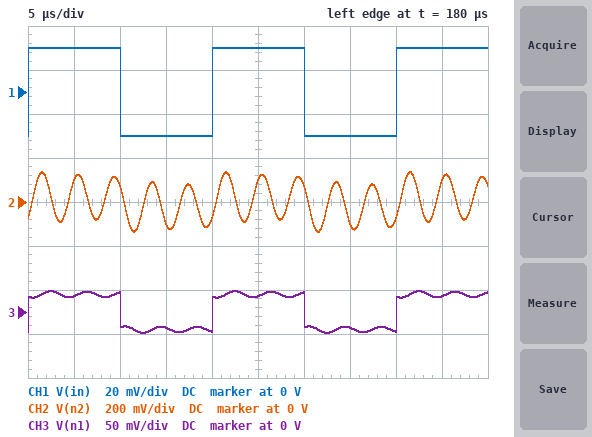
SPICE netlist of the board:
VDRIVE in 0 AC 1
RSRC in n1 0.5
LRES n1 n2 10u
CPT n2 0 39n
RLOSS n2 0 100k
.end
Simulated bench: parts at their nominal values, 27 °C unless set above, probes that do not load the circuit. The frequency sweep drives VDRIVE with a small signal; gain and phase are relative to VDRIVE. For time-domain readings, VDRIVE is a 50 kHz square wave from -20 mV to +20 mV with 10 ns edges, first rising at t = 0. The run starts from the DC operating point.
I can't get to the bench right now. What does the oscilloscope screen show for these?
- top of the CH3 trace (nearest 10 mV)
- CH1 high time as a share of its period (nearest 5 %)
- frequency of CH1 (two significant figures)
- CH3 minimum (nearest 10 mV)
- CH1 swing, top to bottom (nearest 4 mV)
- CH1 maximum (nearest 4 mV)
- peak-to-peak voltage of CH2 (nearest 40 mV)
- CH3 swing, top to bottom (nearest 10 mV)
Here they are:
20 mV
50 %
50 kHz
-20 mV
40 mV
20 mV
280 mV
50 mV
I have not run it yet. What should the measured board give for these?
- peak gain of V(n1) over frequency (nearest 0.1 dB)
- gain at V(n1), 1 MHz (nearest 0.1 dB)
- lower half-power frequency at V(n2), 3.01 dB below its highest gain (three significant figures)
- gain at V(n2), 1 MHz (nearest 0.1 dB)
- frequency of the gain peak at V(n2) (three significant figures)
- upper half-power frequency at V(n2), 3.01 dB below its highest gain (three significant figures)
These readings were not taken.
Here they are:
0 dB
0 dB
251 kHz
-23.2 dB
255 kHz
259 kHz
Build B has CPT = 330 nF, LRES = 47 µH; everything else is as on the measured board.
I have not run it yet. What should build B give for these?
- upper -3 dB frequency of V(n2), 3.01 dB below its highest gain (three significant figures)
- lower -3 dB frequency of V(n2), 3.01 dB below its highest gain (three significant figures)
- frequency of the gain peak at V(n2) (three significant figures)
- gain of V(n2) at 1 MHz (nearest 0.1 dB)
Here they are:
41.2 kHz
39.5 kHz
40.4 kHz
-55.7 dB
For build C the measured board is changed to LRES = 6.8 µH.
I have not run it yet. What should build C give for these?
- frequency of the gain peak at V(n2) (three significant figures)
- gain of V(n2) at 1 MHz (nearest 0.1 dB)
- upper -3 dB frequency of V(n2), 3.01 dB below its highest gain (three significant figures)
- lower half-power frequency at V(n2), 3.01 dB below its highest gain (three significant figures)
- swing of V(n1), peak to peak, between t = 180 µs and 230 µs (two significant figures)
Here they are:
309 kHz
-19.5 dB
315 kHz
303 kHz
42 mV
